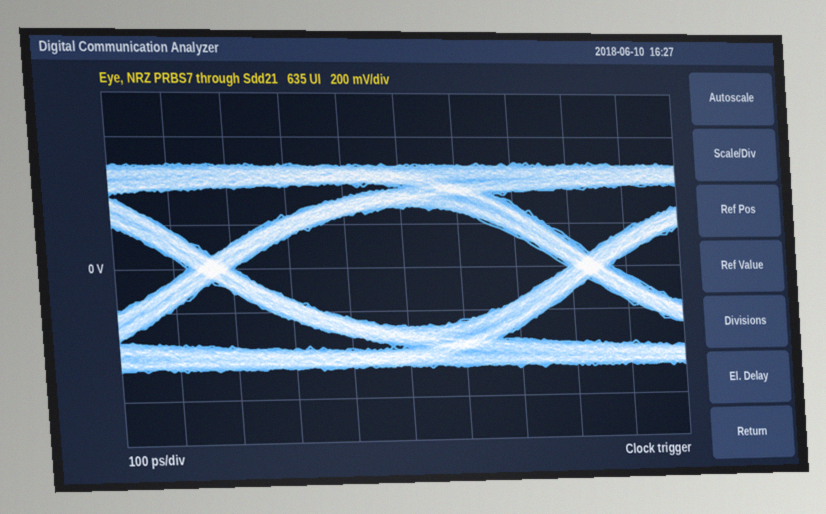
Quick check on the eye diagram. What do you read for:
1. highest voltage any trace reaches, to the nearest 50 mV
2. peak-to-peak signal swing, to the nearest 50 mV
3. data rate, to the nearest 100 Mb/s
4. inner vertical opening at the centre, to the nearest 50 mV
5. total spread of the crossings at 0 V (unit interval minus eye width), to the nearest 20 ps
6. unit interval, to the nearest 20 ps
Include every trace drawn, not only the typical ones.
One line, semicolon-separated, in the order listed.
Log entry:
500 mV; 950 mV; 1.5 Gb/s; 550 mV; 80 ps; 660 ps
